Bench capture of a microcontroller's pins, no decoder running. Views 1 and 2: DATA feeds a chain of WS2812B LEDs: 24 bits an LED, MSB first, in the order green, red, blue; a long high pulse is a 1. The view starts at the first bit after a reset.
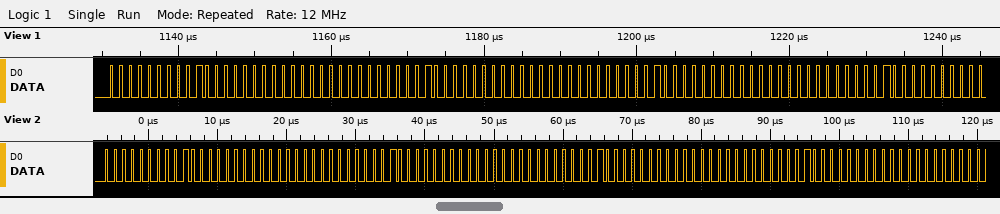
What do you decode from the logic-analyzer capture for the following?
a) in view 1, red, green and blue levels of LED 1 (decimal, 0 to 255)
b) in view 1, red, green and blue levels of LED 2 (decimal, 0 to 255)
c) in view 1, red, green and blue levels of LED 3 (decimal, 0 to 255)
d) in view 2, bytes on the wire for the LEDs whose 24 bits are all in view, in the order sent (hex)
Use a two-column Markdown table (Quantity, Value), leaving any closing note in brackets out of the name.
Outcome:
| Quantity | Value |
|---|---|
| in view 1, red, green and blue levels of LED 1 | 64, 0, 0 |
| in view 1, red, green and blue levels of LED 2 | 64, 0, 0 |
| in view 1, red, green and blue levels of LED 3 | 64, 0, 0 |
| in view 2, bytes on the wire for the LEDs whose 24 bits are all in view, in the order sent | 00 40 00 00 40 00 00 40 00 00 40 00 |
